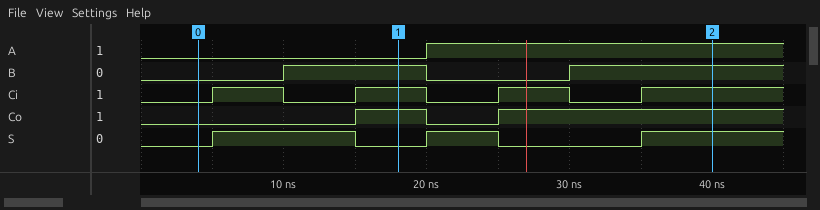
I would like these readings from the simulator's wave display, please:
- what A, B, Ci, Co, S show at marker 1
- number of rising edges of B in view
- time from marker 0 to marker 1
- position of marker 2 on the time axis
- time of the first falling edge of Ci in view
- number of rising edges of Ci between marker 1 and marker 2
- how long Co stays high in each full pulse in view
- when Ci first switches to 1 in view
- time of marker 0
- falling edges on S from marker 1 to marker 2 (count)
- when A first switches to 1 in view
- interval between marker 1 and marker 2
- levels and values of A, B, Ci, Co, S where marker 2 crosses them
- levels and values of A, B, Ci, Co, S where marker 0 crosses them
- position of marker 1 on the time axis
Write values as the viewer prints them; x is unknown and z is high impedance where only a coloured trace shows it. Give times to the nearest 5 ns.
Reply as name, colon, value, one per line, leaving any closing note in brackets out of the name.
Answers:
what A, B, Ci, Co, S show at marker 1: A=0, B=1, Ci=1, Co=1, S=0
number of rising edges of B in view: 2
time from marker 0 to marker 1: 15 ns
position of marker 2 on the time axis: 40 ns
time of the first falling edge of Ci in view: 10 ns
number of rising edges of Ci between marker 1 and marker 2: 2
how long Co stays high in each full pulse in view: 5 ns
when Ci first switches to 1 in view: 5 ns
time of marker 0: 5 ns
falling edges on S from marker 1 to marker 2: 1
when A first switches to 1 in view: 20 ns
interval between marker 1 and marker 2: 20 ns
levels and values of A, B, Ci, Co, S where marker 2 crosses them: A=1, B=1, Ci=1, Co=1, S=1
levels and values of A, B, Ci, Co, S where marker 0 crosses them: A=0, B=0, Ci=0, Co=0, S=0
position of marker 1 on the time axis: 20 ns
